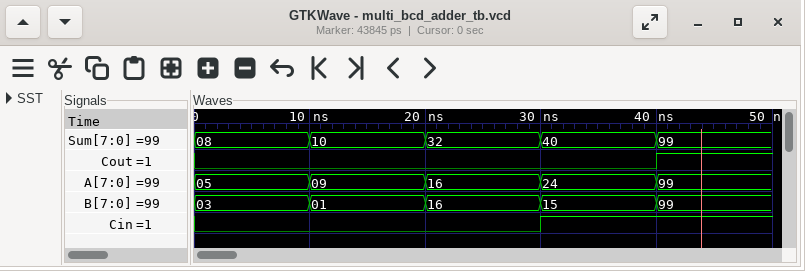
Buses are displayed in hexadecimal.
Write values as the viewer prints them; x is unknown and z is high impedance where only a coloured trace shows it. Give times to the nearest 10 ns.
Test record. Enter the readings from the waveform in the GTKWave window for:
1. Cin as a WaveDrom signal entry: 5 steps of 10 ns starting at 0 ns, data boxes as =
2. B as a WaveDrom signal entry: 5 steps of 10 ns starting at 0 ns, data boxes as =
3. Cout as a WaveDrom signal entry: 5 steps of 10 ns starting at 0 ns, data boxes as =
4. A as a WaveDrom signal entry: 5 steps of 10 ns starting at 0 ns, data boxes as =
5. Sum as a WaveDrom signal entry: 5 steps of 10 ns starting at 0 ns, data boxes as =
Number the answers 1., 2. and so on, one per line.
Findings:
1. {name: 'Cin', wave: '0..1.'}
2. {name: 'B', wave: '=====', data: '03 01 16 15 99'}
3. {name: 'Cout', wave: '0...1'}
4. {name: 'A', wave: '=====', data: '05 09 16 24 99'}
5. {name: 'Sum', wave: '=====', data: '08 10 32 40 99'}
